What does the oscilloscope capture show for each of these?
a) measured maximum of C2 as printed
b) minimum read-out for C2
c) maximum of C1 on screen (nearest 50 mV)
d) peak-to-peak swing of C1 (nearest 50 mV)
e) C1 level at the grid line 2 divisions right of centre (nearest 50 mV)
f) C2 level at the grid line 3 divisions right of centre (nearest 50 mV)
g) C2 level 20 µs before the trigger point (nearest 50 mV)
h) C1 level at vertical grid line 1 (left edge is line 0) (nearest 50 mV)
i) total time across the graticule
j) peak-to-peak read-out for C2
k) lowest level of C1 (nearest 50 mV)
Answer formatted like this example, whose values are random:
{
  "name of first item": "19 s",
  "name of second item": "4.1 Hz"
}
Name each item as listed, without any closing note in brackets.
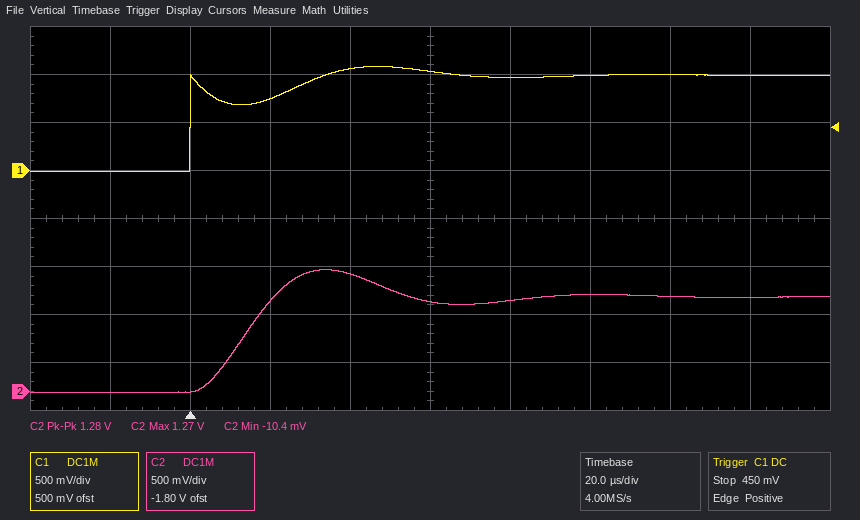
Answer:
{
  "measured maximum of C2 as printed": "1.27 V",
  "minimum read-out for C2": "-10.4 mV",
  "maximum of C1 on screen": "1.10 V",
  "peak-to-peak swing of C1": "1.10 V",
  "C1 level at the grid line 2 divisions right of centre": "1.00 V",
  "C2 level at the grid line 3 divisions right of centre": "1.00 V",
  "C2 level 20 µs before the trigger point": "0 mV",
  "C1 level at vertical grid line 1 (left edge is line 0)": "0 mV",
  "total time across the graticule": "200 µs",
  "peak-to-peak read-out for C2": "1.28 V",
  "lowest level of C1": "0 mV"
}
